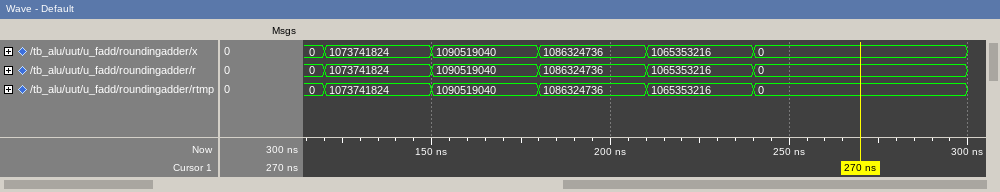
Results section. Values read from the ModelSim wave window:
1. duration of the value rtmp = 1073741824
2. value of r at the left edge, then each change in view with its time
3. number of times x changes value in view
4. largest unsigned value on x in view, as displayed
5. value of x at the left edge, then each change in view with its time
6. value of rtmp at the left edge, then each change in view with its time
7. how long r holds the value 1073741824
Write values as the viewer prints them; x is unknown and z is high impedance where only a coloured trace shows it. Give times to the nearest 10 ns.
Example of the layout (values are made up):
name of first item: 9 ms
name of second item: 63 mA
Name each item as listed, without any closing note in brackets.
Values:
duration of the value rtmp = 1073741824: 30 ns
value of r at the left edge, then each change in view with its time: 0, 1073741824 at 120 ns, 1090519040 at 150 ns, 1086324736 at 180 ns, 1065353216 at 210 ns, 0 at 240 ns
number of times x changes value in view: 5
largest unsigned value on x in view, as displayed: 1090519040
value of x at the left edge, then each change in view with its time: 0, 1073741824 at 120 ns, 1090519040 at 150 ns, 1086324736 at 180 ns, 1065353216 at 210 ns, 0 at 240 ns
value of rtmp at the left edge, then each change in view with its time: 0, 1073741824 at 120 ns, 1090519040 at 150 ns, 1086324736 at 180 ns, 1065353216 at 210 ns, 0 at 240 ns
how long r holds the value 1073741824: 30 ns
